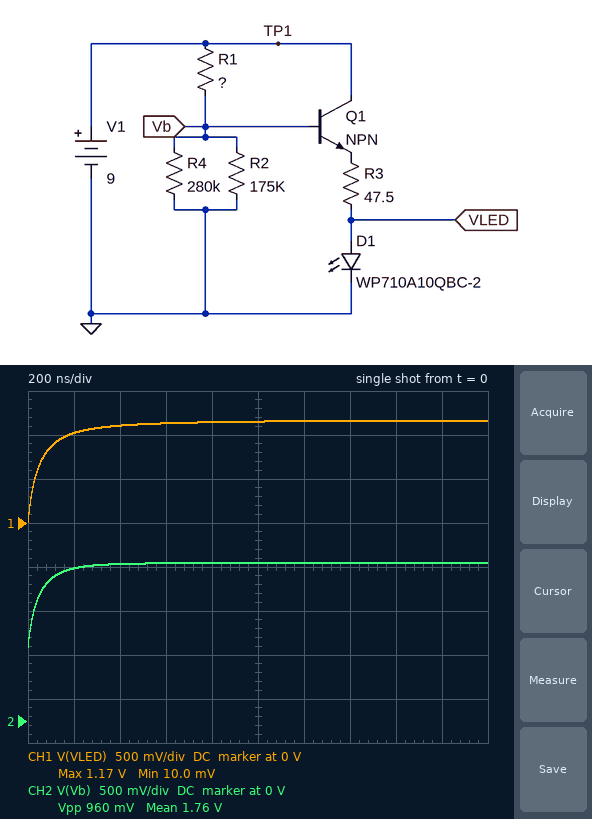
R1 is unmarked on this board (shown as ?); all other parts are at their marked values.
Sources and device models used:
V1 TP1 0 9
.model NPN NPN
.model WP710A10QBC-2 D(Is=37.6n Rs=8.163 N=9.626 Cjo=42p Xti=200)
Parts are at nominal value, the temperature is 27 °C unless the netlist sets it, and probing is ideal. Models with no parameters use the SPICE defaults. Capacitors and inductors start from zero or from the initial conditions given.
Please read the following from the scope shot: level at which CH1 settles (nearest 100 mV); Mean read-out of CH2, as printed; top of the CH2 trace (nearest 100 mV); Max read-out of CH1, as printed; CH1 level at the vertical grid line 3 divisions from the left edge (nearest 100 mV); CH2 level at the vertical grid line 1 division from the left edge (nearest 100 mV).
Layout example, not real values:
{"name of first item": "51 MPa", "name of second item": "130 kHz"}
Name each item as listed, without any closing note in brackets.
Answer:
{"level at which CH1 settles": "1.2 V", "Mean read-out of CH2, as printed": "1.76 V", "top of the CH2 trace": "1.8 V", "Max read-out of CH1, as printed": "1.17 V", "CH1 level at the vertical grid line 3 divisions from the left edge": "1.1 V", "CH2 level at the vertical grid line 1 division from the left edge": "1.7 V"}
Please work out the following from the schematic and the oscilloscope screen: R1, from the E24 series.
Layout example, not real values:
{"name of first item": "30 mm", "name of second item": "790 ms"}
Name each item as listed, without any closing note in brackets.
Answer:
{"R1, from the E24 series": "430 kΩ"}
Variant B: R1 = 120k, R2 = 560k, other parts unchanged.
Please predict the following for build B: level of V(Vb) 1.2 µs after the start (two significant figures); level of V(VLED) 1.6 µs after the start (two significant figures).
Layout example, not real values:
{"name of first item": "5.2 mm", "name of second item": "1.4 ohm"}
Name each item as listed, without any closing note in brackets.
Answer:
{"level of V(Vb) 1.2 µs after the start": "3.7 V", "level of V(VLED) 1.6 µs after the start": "2.8 V"}
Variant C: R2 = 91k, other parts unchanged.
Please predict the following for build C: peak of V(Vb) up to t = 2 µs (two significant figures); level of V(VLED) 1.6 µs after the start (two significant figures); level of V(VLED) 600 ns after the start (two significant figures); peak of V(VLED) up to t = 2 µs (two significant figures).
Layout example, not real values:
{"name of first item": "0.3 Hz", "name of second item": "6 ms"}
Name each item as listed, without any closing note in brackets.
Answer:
{"peak of V(Vb) up to t = 2 µs": "1.2 V", "level of V(VLED) 1.6 µs after the start": "630 mV", "level of V(VLED) 600 ns after the start": "600 mV", "peak of V(VLED) up to t = 2 µs": "640 mV"}
